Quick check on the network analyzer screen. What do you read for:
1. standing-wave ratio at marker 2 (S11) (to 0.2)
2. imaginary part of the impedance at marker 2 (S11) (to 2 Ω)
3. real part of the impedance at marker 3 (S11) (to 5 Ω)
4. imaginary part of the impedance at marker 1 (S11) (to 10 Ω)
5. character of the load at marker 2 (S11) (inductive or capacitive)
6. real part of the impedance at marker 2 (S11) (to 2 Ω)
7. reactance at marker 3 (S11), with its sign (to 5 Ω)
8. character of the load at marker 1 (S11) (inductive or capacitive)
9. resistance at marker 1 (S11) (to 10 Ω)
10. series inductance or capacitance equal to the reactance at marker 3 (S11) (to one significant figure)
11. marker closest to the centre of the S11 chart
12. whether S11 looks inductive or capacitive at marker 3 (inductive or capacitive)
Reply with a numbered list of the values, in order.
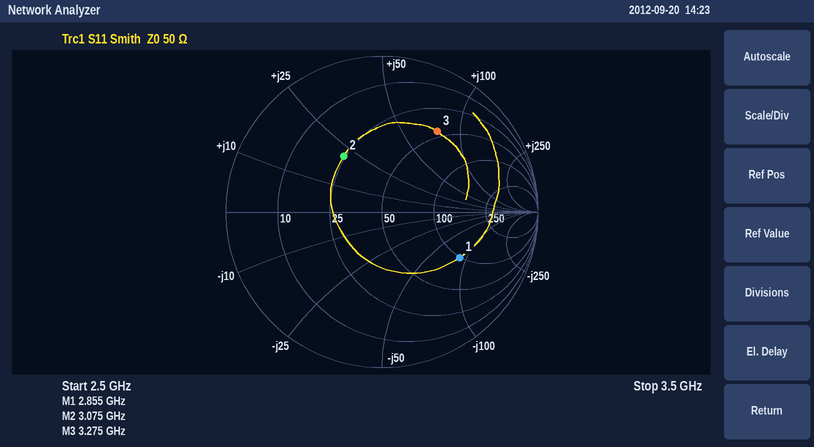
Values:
1. 2.6
2. +22 Ω
3. 45 Ω
4. -90 Ω
5. inductive
6. 24 Ω
7. +75 Ω
8. capacitive
9. 100 Ω
10. 4 nH
11. marker 2
12. inductive
